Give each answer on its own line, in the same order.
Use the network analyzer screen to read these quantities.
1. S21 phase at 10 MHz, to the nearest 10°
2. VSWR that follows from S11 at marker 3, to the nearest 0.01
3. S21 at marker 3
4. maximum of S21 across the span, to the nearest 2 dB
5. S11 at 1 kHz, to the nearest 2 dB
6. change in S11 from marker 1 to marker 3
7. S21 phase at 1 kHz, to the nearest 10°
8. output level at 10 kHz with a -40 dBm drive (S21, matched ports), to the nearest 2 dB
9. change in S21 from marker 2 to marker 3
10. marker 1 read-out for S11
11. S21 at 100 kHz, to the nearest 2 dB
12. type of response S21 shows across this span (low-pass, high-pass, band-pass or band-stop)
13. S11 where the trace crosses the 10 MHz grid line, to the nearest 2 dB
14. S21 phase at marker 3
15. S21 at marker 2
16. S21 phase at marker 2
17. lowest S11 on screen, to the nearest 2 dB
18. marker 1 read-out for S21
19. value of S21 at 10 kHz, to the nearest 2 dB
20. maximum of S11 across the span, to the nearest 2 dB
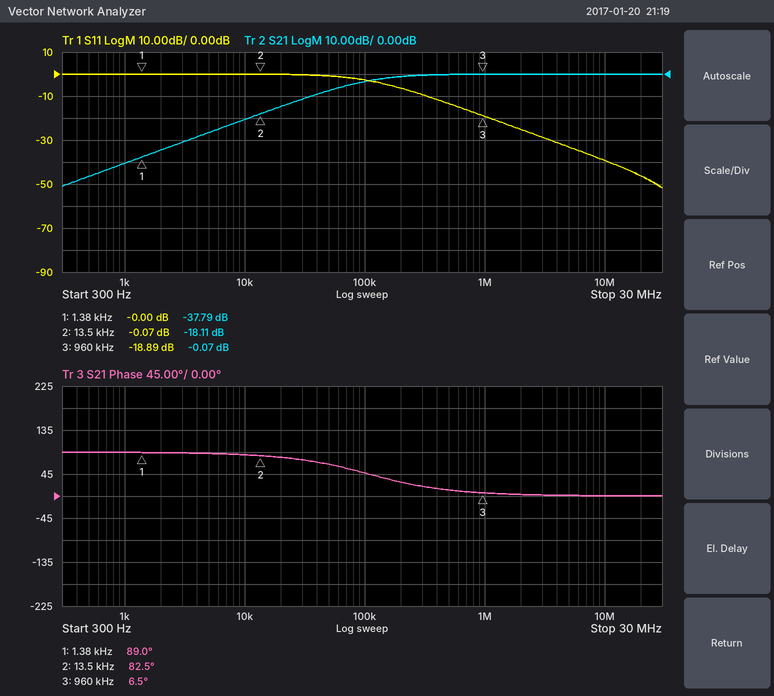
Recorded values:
0°
1.26
-0.07 dB
0 dB
0 dB
-18.89 dB
90°
-60 dBm
18.04 dB
-0.00 dB
-4 dB
high-pass
-40 dB
6.5°
-18.11 dB
82.5°
-52 dB
-37.79 dB
-20 dB
0 dB
